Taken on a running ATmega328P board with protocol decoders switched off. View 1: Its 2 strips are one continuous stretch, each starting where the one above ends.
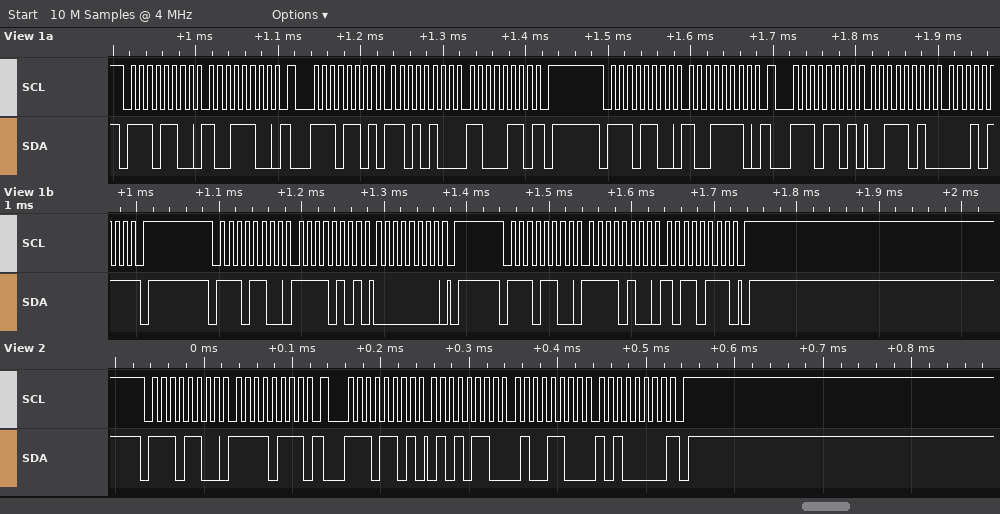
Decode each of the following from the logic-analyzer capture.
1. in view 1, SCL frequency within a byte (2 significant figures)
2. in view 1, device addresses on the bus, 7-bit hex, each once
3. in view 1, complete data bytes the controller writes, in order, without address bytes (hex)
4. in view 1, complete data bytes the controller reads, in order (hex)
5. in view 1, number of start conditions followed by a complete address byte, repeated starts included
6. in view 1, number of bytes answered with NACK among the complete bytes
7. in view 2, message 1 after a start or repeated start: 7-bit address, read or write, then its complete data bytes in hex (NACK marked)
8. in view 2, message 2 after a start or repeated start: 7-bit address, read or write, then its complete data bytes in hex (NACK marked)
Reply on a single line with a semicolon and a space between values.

100 kHz; 0x76; 9C 9E F5 00 F4 B7; D4 C6 3A 17; 6; 2; 0x76 write: F7; 0x76 read: 56 4C A0 NACK
